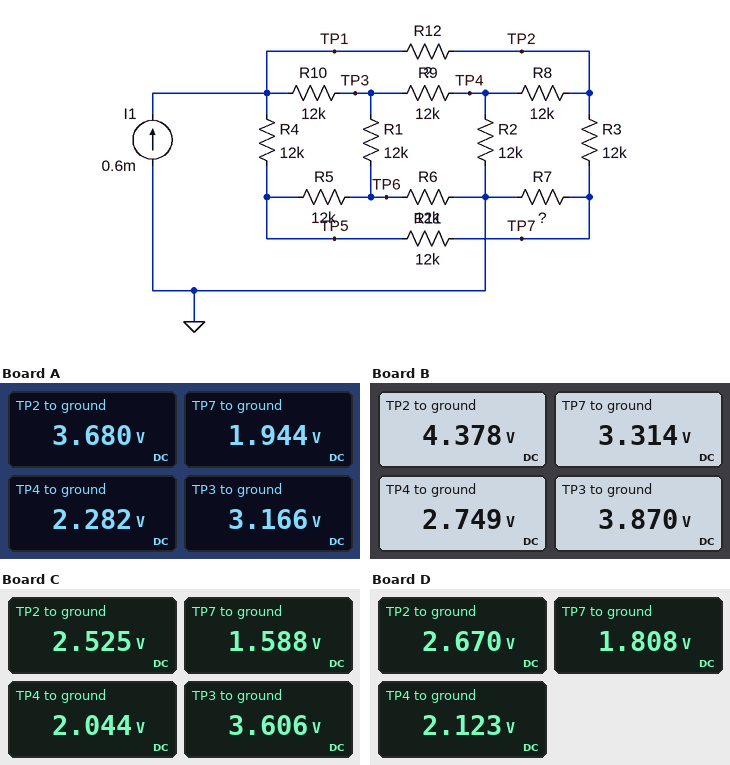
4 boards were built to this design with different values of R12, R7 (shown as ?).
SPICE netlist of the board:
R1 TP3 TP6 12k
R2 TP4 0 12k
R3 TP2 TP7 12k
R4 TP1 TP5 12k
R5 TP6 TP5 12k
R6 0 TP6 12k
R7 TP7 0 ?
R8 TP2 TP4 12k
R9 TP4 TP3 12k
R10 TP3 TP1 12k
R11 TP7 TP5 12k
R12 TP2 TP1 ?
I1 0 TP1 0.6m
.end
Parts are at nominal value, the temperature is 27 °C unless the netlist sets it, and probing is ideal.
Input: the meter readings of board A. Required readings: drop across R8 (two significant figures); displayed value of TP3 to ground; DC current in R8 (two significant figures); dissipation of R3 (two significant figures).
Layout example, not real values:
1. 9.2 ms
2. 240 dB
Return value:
1. 1.4 V
2. 3.166 V
3. 120 µA
4. 250 µW
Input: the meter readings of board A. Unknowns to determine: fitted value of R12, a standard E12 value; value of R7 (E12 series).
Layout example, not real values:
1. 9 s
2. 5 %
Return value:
1. 5.6 kΩ
2. 8.2 kΩ
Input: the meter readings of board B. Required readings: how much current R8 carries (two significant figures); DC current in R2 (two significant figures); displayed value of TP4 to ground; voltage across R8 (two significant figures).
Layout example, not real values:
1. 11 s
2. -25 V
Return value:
1. 140 µA
2. 230 µA
3. 2.749 V
4. 1.6 V
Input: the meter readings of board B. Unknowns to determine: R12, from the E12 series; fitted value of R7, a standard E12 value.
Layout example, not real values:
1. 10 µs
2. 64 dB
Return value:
1. 8.2 kΩ
2. 22 kΩ
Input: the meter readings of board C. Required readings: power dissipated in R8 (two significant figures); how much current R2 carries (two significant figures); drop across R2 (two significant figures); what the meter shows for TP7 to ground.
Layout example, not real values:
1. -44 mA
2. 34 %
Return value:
1. 19 µW
2. 170 µA
3. 2.0 V
4. 1.588 V
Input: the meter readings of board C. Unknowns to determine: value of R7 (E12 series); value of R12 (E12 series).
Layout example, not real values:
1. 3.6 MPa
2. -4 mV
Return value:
1. 6.8 kΩ
2. 33 kΩ
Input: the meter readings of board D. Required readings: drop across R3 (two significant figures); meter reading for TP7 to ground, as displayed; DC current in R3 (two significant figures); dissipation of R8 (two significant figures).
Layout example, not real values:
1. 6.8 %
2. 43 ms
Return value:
1. 860 mV
2. 1.808 V
3. 72 µA
4. 25 µW
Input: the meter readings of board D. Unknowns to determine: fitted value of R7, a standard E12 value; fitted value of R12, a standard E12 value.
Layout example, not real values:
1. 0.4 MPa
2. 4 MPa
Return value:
1. 8.2 kΩ
2. 33 kΩ
